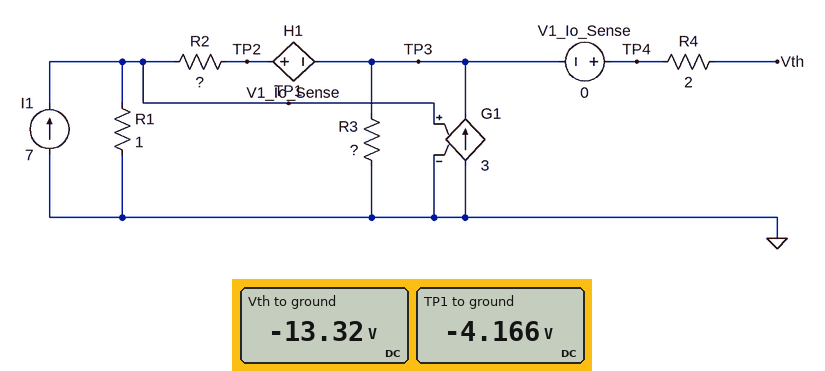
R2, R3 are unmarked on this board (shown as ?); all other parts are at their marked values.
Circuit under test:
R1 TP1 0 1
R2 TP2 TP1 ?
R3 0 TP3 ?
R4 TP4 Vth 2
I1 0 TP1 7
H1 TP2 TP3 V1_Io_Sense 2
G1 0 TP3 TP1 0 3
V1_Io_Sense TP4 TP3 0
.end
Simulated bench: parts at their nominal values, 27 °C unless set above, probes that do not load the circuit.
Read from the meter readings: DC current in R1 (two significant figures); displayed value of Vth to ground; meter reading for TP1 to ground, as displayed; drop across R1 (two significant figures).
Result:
4.2 A
-13.32 V
-4.166 V
4.2 V
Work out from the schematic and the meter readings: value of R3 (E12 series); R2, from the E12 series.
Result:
10 Ω
0.82 Ω
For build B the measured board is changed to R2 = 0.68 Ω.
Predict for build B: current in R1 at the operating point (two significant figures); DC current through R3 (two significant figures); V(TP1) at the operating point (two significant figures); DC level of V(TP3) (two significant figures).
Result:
4.1 A
1.2 A
-4.1 V
-12 V
